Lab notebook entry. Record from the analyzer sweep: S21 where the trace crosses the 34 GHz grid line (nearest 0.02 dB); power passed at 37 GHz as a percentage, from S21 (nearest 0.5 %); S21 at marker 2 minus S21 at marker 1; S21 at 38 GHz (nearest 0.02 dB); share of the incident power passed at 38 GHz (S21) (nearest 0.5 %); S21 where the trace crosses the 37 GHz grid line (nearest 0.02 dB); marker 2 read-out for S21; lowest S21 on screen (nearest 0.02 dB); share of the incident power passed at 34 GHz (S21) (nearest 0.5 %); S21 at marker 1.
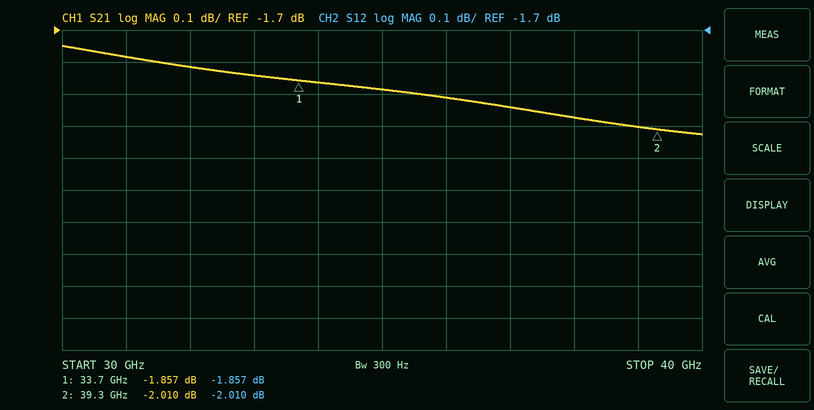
-1.86 dB
64.0 %
-0.153 dB
-1.98 dB
63.5 %
-1.94 dB
-2.010 dB
-2.02 dB
65.0 %
-1.857 dB
